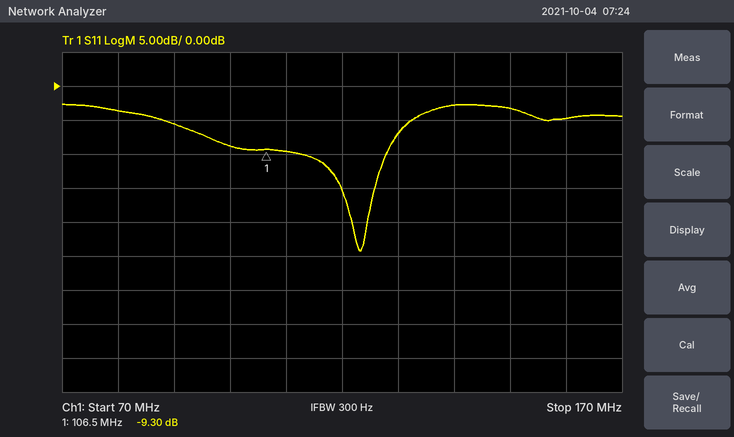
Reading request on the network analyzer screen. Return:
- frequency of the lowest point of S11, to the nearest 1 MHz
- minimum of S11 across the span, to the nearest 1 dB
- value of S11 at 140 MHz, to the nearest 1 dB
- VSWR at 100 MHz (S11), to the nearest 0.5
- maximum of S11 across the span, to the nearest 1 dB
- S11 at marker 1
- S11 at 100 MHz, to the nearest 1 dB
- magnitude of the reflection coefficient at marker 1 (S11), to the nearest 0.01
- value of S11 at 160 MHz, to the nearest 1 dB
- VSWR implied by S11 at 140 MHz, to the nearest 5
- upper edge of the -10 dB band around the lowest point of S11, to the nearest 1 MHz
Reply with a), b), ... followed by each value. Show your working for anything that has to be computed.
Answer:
a) 123 MHz
b) -24 dB
c) -3 dB
d) |Γ| = 10^(-9/20) = 0.3548; VSWR = (1 + 0.3548)/(1 − 0.3548) ≈ 2.10, so 2.0 to the nearest 0.5
e) -3 dB
f) -9.30 dB
g) -9 dB
h) 10^(-9.3/20) ≈ 0.34
i) -5 dB
j) |Γ| = 10^(-3/20) = 0.7079; VSWR = (1 + 0.7079)/(1 − 0.7079) ≈ 5.85, so 5 to the nearest 5
k) 128 MHz
